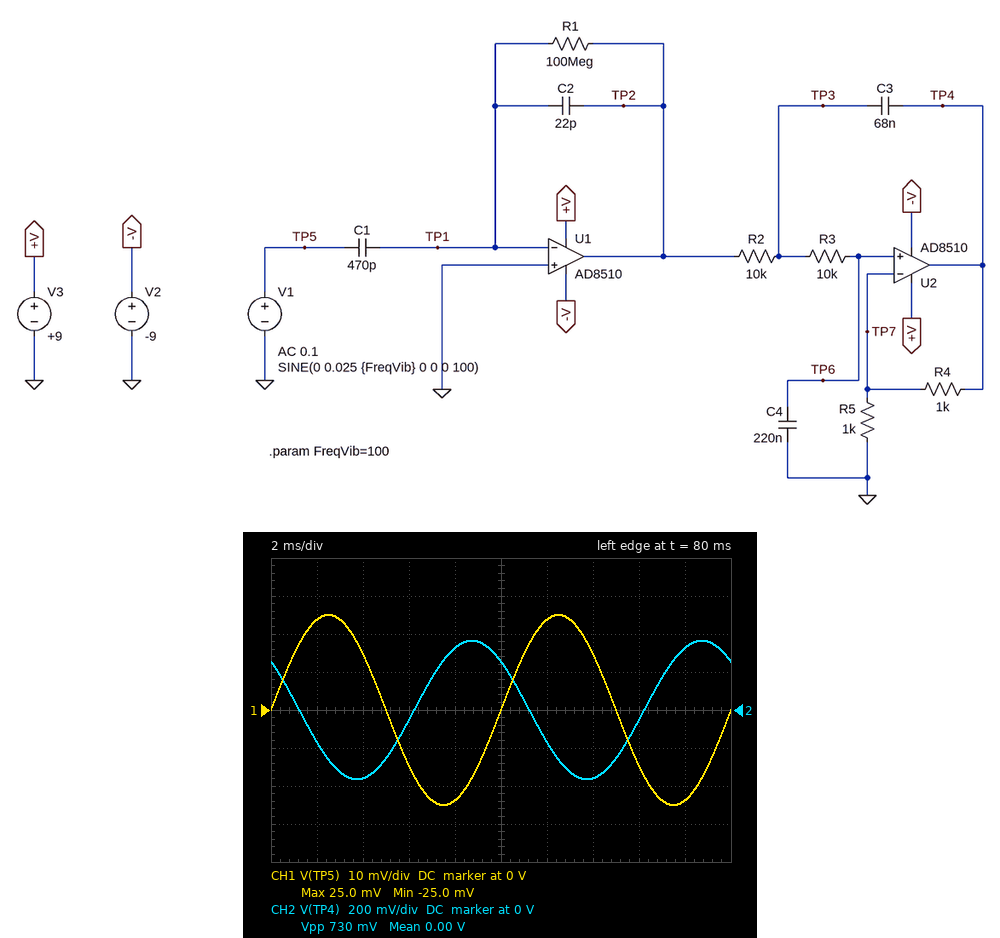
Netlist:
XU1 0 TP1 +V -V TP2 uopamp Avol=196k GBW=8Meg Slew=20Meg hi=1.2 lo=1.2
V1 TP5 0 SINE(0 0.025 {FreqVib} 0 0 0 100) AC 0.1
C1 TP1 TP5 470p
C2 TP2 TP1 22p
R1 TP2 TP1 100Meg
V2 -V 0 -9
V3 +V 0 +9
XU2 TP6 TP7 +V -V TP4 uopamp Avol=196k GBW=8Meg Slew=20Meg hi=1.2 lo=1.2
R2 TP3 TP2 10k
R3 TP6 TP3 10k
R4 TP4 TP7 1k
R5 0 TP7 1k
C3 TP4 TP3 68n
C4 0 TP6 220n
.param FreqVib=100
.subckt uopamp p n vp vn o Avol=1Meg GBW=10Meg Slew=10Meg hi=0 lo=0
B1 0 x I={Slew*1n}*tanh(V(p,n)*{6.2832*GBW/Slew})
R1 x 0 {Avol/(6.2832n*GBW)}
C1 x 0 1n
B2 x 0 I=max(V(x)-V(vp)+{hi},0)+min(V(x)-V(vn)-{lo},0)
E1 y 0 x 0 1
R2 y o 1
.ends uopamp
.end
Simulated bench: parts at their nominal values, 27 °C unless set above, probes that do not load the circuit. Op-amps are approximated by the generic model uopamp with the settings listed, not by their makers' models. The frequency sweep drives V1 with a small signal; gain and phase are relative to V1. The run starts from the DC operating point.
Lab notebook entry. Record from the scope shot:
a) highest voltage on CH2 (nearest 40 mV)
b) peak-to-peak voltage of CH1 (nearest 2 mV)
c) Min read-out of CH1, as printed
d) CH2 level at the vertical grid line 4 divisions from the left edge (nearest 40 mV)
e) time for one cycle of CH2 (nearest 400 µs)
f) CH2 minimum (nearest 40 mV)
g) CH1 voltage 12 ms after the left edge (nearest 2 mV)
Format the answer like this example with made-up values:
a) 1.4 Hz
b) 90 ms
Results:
a) 360 mV
b) 50 mV
c) -25.0 mV
d) 320 mV
e) 10.0 ms
f) -360 mV
g) 24 mV
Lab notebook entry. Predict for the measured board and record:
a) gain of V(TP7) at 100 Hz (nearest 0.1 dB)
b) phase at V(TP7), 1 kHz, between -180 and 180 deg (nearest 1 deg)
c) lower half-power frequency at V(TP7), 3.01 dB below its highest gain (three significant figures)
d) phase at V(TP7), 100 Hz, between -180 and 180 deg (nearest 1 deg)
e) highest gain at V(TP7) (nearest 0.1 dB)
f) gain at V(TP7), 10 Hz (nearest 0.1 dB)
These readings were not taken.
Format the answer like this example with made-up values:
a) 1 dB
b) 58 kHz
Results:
a) 17.3 dB
b) 26 deg
c) 23.9 Hz
d) 136 deg
e) 18.6 dB
f) 9.1 dB
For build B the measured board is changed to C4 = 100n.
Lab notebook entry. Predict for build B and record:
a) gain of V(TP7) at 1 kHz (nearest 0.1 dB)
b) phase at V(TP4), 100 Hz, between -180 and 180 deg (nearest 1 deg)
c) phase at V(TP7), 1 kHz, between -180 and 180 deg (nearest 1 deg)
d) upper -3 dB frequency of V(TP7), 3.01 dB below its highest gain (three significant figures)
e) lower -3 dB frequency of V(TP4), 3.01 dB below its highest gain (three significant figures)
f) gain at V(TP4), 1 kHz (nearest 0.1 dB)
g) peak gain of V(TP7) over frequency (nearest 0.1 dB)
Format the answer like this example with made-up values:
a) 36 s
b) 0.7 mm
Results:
a) -2.1 dB
b) 167 deg
c) 22 deg
d) 217 Hz
e) 45.1 Hz
f) 3.9 dB
g) 23.9 dB
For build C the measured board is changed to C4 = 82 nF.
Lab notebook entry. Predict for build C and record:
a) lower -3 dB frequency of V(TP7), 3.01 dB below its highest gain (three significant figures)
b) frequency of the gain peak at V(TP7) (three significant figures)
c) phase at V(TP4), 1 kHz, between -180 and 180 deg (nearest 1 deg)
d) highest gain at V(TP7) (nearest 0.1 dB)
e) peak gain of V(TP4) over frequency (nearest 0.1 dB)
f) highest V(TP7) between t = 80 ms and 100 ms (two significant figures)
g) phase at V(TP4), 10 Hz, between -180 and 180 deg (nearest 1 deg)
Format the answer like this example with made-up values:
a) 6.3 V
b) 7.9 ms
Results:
a) 55.9 Hz
b) 140 Hz
c) 20 deg
d) 25.4 dB
e) 31.4 dB
f) 440 mV
g) -101 deg
